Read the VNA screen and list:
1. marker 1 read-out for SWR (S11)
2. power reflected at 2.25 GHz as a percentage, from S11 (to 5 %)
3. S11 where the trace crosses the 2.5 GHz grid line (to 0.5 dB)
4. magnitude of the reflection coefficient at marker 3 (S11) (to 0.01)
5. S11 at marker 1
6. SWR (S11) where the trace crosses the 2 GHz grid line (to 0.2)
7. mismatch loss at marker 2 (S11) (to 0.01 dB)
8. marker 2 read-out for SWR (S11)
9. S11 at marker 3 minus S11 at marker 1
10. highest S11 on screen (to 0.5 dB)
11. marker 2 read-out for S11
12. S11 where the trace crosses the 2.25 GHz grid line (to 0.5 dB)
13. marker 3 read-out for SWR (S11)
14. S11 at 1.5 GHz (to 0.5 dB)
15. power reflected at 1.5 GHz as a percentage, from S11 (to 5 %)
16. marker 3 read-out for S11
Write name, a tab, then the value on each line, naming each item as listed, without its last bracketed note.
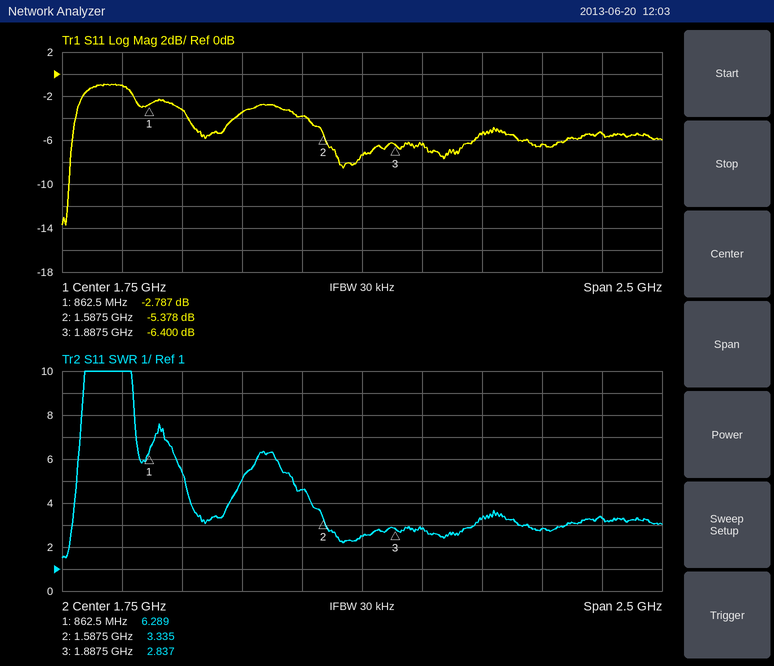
marker 1 read-out for SWR	6.289
power reflected at 2.25 GHz as a percentage, from S11	30 %
S11 where the trace crosses the 2.5 GHz grid line	-6.5 dB
magnitude of the reflection coefficient at marker 3 (S11)	0.48
S11 at marker 1	-2.787 dB
SWR (S11) where the trace crosses the 2 GHz grid line	2.8
mismatch loss at marker 2 (S11)	1.49 dB
marker 2 read-out for SWR	3.335
S11 at marker 3 minus S11 at marker 1	-3.613 dB
highest S11 on screen	-1.0 dB
marker 2 read-out for S11	-5.378 dB
S11 where the trace crosses the 2.25 GHz grid line	-5.5 dB
marker 3 read-out for SWR	2.837
S11 at 1.5 GHz	-4.0 dB
power reflected at 1.5 GHz as a percentage, from S11	40 %
marker 3 read-out for S11	-6.400 dB
